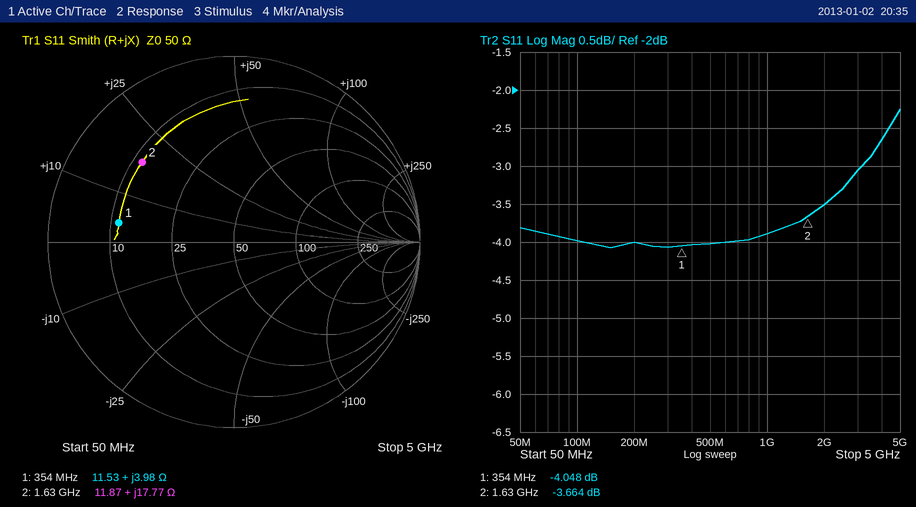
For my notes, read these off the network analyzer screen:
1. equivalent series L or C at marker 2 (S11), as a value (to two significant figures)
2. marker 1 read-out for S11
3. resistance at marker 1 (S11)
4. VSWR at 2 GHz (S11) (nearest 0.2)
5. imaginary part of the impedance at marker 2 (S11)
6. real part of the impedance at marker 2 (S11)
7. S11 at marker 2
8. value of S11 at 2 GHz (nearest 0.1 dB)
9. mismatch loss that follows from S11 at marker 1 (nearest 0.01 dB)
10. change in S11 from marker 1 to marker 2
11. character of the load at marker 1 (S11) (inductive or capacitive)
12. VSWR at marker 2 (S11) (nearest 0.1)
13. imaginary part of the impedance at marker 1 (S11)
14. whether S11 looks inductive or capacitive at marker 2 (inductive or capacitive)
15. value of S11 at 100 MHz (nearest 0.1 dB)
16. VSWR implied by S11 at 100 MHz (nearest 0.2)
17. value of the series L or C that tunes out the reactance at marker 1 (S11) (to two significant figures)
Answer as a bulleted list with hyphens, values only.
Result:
- 1.7 nH
- -4.048 dB
- 11.53 Ω
- 5.0
- +17.77 Ω
- 11.87 Ω
- -3.664 dB
- -3.5 dB
- 2.17 dB
- 0.384 dB
- inductive
- 4.8
- +3.98 Ω
- inductive
- -4.0 dB
- 4.4
- 110 pF
